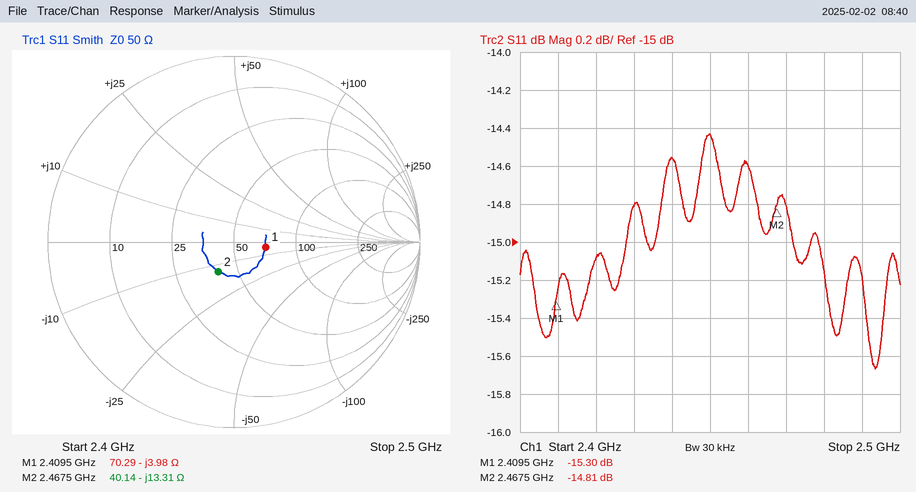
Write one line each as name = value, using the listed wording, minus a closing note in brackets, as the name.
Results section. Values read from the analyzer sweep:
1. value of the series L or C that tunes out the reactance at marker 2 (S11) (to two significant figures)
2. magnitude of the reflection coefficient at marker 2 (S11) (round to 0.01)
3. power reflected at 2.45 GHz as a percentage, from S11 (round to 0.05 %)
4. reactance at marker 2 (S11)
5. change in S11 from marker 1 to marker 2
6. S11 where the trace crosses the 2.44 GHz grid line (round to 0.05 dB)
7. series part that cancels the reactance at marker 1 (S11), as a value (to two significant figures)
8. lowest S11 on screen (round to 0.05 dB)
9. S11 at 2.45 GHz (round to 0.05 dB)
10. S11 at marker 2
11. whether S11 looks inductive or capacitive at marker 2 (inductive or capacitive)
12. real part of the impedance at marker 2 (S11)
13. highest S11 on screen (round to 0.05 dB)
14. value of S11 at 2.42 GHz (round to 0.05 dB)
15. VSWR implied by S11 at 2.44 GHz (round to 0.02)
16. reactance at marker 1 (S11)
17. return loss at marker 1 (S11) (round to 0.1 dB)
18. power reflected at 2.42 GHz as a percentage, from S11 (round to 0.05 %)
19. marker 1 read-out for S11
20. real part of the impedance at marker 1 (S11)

value of the series L or C that tunes out the reactance at marker 2 (S11) = 860 pH
magnitude of the reflection coefficient at marker 2 (S11) = 0.18
power reflected at 2.45 GHz as a percentage, from S11 = 3.60 %
reactance at marker 2 = -13.31 Ω
change in S11 from marker 1 to marker 2 = 0.49 dB
S11 where the trace crosses the 2.44 GHz grid line = -14.55 dB
series part that cancels the reactance at marker 1 (S11), as a value = 260 pH
lowest S11 on screen = -15.65 dB
S11 at 2.45 GHz = -14.45 dB
S11 at marker 2 = -14.81 dB
whether S11 looks inductive or capacitive at marker 2 = capacitive
real part of the impedance at marker 2 = 40.14 Ω
highest S11 on screen = -14.45 dB
value of S11 at 2.42 GHz = -15.10 dB
VSWR implied by S11 at 2.44 GHz = 1.46
reactance at marker 1 = -3.98 Ω
return loss at marker 1 (S11) = 15.3 dB
power reflected at 2.42 GHz as a percentage, from S11 = 3.10 %
marker 1 read-out for S11 = -15.30 dB
real part of the impedance at marker 1 = 70.29 Ω
